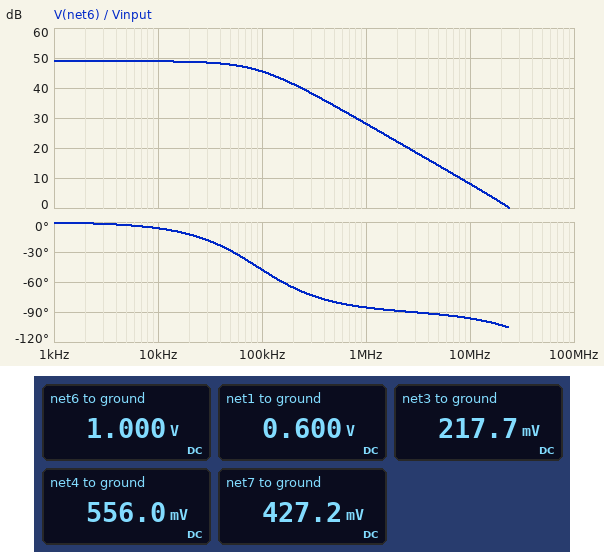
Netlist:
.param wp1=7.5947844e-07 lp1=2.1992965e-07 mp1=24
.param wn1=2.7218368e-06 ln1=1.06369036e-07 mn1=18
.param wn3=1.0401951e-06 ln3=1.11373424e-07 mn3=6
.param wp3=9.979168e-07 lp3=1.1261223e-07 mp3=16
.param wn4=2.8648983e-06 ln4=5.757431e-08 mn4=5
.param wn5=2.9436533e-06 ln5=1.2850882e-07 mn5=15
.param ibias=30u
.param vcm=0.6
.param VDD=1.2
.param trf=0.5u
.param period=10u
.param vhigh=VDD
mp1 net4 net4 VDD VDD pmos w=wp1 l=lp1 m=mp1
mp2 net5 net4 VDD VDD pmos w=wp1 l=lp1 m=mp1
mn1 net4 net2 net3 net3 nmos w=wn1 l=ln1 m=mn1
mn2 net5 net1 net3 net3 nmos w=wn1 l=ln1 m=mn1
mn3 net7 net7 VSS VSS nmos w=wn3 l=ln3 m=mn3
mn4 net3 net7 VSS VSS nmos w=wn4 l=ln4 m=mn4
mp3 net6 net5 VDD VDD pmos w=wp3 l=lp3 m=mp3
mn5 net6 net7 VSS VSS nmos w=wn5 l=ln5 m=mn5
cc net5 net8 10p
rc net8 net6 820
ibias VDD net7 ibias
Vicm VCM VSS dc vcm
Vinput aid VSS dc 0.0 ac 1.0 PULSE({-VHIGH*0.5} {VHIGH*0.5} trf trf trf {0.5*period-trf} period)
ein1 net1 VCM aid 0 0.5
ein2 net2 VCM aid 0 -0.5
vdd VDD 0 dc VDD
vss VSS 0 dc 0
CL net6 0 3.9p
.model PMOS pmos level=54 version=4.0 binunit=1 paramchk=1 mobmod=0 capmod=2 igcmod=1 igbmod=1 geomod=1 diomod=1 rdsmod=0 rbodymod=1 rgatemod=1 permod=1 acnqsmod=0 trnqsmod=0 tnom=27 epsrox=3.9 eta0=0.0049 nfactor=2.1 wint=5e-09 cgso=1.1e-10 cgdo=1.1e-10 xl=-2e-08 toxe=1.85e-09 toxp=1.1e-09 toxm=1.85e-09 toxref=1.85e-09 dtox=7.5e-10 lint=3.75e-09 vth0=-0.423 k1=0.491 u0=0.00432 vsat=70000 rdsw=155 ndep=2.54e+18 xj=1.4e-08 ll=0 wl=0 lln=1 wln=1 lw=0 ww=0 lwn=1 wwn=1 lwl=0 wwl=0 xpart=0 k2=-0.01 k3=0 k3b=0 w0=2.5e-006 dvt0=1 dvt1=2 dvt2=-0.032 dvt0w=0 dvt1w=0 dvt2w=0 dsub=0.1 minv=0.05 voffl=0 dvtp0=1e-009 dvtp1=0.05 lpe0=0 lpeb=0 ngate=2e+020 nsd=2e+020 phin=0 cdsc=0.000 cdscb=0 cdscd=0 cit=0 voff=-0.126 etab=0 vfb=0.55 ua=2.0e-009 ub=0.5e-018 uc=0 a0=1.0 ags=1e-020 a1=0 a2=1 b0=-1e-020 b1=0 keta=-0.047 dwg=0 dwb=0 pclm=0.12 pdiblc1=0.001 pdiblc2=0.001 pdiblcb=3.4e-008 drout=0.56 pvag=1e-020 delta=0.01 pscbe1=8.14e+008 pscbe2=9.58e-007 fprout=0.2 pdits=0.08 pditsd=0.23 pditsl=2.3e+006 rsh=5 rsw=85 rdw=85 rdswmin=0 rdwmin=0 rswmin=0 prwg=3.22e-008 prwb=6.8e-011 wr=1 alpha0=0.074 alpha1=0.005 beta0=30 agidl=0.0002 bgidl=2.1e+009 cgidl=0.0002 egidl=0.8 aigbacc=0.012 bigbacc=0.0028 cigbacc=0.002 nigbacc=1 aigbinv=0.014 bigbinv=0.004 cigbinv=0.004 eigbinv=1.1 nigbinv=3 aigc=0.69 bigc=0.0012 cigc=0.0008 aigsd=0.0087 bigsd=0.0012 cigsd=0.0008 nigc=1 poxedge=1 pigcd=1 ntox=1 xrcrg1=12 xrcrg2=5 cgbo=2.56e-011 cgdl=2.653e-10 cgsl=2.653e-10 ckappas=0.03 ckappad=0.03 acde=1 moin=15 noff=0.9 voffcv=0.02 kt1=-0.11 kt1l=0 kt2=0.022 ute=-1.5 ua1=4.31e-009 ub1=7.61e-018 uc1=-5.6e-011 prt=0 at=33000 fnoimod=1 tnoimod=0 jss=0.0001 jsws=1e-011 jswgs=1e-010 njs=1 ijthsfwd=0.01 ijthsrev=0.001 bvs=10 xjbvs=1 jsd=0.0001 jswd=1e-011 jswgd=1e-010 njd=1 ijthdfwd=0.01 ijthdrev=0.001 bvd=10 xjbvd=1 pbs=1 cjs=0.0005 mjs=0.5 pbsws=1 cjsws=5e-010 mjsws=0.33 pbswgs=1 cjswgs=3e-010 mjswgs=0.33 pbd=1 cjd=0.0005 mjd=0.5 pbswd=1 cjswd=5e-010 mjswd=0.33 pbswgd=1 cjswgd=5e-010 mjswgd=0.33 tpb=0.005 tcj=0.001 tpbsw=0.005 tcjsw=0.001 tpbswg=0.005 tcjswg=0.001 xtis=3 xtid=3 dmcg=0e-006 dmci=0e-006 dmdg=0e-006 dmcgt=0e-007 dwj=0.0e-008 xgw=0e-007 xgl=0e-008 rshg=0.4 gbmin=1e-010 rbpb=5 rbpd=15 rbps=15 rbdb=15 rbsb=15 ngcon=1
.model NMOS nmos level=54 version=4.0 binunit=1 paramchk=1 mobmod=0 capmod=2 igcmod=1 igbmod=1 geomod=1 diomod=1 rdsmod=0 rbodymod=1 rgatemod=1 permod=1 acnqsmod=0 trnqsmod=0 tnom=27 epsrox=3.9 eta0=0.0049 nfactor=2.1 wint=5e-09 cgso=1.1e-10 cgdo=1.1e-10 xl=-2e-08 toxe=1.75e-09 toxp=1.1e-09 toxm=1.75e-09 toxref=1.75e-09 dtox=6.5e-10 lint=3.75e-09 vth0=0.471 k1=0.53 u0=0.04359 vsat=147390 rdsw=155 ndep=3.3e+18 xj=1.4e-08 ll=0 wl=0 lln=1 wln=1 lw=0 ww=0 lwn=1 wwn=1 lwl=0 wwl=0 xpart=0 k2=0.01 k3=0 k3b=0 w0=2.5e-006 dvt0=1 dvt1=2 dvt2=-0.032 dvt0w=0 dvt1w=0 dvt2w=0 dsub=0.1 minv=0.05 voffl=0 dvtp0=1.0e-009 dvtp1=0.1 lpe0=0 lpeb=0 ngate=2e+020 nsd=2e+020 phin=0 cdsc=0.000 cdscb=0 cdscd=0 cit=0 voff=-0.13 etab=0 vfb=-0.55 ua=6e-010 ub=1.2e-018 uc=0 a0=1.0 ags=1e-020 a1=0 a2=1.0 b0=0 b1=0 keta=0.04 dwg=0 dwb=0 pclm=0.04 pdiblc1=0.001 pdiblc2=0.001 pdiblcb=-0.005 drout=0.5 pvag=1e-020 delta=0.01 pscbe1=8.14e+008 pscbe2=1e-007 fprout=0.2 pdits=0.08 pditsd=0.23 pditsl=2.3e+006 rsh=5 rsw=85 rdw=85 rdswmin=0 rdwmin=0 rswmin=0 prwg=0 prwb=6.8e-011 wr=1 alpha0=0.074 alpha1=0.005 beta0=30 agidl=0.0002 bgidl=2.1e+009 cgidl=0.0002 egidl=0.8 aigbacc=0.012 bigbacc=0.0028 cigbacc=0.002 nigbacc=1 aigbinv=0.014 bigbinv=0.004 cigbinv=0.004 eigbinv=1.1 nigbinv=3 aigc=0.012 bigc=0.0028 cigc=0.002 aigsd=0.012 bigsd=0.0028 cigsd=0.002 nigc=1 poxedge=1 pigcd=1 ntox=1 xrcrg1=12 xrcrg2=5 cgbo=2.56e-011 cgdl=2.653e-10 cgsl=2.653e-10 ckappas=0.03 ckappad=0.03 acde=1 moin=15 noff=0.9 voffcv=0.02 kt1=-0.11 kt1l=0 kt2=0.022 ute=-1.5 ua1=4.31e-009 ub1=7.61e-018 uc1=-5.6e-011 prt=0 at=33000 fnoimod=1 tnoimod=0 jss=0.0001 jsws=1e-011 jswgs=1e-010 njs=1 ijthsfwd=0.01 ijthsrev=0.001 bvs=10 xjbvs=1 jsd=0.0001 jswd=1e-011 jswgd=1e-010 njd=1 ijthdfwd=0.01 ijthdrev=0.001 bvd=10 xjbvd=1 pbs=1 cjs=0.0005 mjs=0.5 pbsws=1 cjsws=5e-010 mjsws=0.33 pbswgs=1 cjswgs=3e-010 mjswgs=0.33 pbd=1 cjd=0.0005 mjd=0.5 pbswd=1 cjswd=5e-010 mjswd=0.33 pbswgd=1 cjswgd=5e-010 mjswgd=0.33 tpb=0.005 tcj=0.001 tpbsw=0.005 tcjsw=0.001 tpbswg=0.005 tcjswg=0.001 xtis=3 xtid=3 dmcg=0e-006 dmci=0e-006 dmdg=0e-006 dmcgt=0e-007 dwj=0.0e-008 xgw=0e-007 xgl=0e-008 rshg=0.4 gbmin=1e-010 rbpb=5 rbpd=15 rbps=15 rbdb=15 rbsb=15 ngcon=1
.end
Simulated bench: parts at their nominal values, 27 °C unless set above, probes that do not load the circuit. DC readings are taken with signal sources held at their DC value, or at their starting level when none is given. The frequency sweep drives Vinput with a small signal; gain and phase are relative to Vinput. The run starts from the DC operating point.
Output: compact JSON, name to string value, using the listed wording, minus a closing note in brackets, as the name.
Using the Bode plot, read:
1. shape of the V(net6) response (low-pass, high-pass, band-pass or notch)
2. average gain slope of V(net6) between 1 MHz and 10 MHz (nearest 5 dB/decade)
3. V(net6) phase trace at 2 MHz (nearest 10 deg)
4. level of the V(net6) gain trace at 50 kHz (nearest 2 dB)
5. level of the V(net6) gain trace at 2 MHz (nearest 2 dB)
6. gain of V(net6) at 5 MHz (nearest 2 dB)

{"shape of the V(net6) response": "low-pass", "average gain slope of V(net6) between 1 MHz and 10 MHz": "-20 dB/decade", "V(net6) phase trace at 2 MHz": "-90 deg", "level of the V(net6) gain trace at 50 kHz": "48 dB", "level of the V(net6) gain trace at 2 MHz": "22 dB", "gain of V(net6) at 5 MHz": "14 dB"}
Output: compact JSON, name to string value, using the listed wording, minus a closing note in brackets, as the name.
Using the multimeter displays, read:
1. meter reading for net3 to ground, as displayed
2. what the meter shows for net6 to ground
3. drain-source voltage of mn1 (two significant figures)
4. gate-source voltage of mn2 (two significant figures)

{"meter reading for net3 to ground, as displayed": "217.7 mV", "what the meter shows for net6 to ground": "1.000 V", "drain-source voltage of mn1": "340 mV", "gate-source voltage of mn2": "380 mV"}
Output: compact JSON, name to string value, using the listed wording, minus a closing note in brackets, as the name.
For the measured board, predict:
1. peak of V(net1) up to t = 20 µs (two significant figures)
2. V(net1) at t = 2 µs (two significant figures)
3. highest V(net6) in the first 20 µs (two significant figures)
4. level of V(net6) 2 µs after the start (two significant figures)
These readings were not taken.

{"peak of V(net1) up to t = 20 µs": "900 mV", "V(net1) at t = 2 µs": "900 mV", "highest V(net6) in the first 20 µs": "1.2 V", "level of V(net6) 2 µs after the start": "1.2 V"}
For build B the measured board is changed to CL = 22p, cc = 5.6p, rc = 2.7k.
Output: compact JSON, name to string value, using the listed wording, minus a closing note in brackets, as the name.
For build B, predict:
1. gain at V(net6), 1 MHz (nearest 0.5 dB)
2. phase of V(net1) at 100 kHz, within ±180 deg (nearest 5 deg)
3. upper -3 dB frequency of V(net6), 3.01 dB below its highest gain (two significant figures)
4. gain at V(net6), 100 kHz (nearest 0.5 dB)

{"gain at V(net6), 1 MHz": "32.5 dB", "phase of V(net1) at 100 kHz, within ±180 deg": "0 deg", "upper -3 dB frequency of V(net6), 3.01 dB below its highest gain": "150 kHz", "gain at V(net6), 100 kHz": "47.5 dB"}
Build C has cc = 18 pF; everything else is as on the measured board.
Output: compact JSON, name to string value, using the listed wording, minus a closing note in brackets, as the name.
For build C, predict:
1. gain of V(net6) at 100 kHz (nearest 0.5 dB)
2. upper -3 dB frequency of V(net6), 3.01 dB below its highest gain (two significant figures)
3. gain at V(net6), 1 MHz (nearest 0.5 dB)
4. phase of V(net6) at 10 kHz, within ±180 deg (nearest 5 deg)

{"gain of V(net6) at 100 kHz": "42.0 dB", "upper -3 dB frequency of V(net6), 3.01 dB below its highest gain": "51 kHz", "gain at V(net6), 1 MHz": "23.0 dB", "phase of V(net6) at 10 kHz, within ±180 deg": "-10 deg"}
